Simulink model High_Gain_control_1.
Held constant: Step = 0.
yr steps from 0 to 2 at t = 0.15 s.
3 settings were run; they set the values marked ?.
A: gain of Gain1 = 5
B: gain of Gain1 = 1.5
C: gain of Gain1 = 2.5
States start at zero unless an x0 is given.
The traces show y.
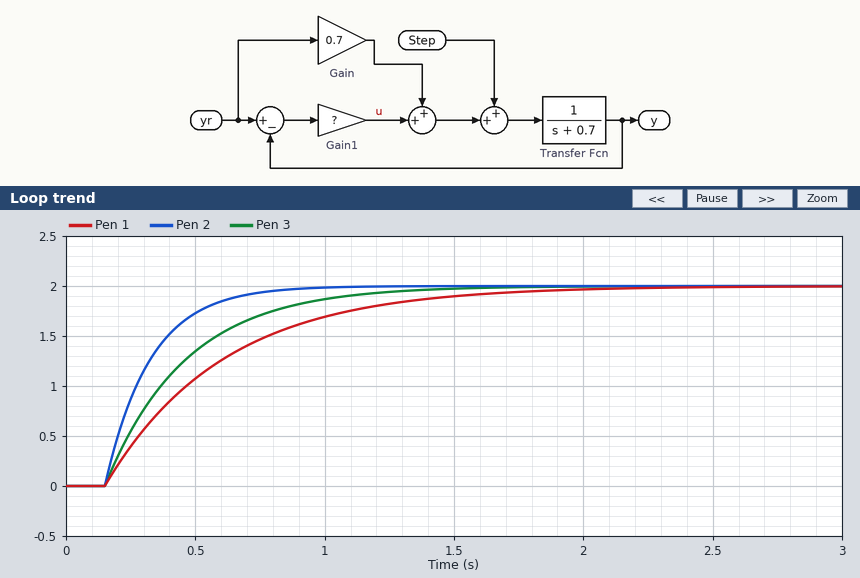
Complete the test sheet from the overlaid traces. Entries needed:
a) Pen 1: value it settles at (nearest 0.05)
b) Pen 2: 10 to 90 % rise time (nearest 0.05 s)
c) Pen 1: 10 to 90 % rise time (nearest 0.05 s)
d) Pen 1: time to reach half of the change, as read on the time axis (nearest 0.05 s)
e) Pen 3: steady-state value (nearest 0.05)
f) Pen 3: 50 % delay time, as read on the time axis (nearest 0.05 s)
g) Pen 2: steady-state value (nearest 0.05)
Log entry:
2.00
0.40 s
1.00 s
0.45 s
2.00
0.35 s
2.00
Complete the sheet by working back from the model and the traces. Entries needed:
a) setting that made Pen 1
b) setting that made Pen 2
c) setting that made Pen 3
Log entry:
B
A
C
